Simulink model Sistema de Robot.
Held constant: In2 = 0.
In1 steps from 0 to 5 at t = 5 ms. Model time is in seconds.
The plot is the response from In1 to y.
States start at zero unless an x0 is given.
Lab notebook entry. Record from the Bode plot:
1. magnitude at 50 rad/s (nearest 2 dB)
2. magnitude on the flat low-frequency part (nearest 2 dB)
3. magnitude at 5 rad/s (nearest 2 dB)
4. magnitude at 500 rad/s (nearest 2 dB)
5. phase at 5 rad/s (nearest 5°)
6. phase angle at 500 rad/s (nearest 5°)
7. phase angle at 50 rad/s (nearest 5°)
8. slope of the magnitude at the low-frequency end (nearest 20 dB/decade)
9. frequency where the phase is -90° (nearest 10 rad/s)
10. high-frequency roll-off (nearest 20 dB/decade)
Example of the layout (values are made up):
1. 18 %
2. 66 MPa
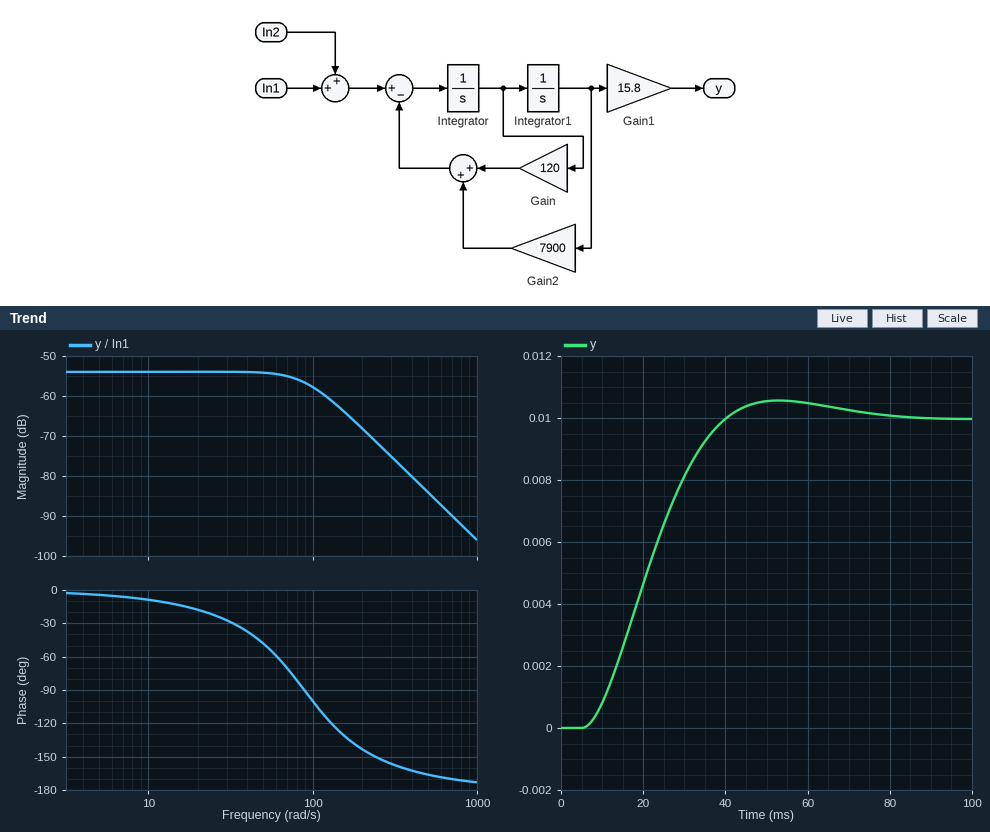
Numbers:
1. -54 dB
2. -54 dB
3. -54 dB
4. -84 dB
5. -5°
6. -165°
7. -50°
8. 0 dB/decade
9. 90 rad/s
10. -40 dB/decade
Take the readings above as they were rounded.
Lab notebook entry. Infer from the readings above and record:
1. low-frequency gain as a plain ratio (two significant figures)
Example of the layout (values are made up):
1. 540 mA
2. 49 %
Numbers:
1. 0.0020
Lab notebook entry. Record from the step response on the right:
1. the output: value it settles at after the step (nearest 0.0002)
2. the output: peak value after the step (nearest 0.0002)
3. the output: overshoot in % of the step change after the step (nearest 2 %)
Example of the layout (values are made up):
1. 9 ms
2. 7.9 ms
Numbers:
1. 0.0100
2. 0.0106
3. 6 %
